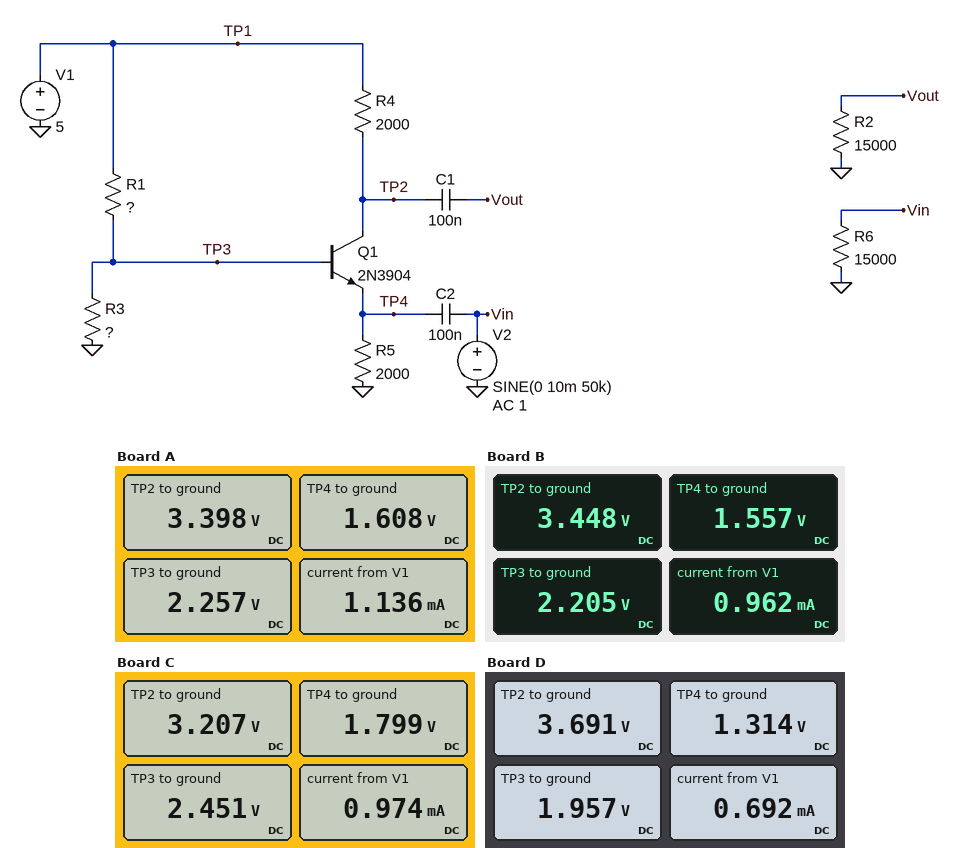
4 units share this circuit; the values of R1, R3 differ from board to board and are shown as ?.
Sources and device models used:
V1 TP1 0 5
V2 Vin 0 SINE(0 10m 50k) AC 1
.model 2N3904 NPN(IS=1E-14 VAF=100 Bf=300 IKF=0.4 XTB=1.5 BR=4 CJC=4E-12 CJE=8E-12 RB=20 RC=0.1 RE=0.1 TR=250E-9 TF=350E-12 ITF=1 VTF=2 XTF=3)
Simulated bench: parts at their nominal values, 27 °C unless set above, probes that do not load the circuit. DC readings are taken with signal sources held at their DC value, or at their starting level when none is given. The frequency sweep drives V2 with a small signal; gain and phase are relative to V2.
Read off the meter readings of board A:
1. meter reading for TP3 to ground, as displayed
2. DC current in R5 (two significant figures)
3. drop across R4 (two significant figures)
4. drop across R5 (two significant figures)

2.257 V
800 µA
1.6 V
1.6 V
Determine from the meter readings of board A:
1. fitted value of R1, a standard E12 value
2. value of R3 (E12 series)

8.2 kΩ
6.8 kΩ
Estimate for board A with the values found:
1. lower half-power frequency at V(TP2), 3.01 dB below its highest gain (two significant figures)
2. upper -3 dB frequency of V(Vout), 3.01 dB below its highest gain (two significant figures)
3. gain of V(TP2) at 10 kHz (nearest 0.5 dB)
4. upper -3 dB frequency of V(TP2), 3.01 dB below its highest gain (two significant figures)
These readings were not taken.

32 kHz
350 kHz
20.5 dB
350 kHz
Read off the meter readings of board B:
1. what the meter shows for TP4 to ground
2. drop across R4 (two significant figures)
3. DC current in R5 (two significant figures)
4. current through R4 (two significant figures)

1.557 V
1.6 V
780 µA
780 µA
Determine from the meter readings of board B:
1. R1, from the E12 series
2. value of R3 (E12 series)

15 kΩ
12 kΩ
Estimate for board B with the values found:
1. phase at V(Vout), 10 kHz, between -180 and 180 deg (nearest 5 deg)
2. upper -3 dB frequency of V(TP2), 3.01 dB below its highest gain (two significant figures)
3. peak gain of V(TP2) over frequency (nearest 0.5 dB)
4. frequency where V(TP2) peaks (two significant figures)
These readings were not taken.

70 deg
250 kHz
30.0 dB
81 kHz
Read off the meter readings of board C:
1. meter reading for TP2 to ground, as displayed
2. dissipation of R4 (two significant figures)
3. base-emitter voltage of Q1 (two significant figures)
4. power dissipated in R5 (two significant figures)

3.207 V
1.6 mW
650 mV
1.6 mW
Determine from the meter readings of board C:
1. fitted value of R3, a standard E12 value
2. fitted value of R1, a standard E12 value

33 kΩ
33 kΩ
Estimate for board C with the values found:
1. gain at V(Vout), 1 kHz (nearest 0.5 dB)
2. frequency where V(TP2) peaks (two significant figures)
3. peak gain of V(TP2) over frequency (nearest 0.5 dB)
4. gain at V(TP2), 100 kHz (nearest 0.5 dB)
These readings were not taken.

0.5 dB
50 kHz
26.0 dB
25.0 dB
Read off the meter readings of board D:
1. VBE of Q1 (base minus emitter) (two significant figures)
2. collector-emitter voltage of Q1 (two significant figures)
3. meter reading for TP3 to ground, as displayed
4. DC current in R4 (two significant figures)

640 mV
2.4 V
1.957 V
650 µA
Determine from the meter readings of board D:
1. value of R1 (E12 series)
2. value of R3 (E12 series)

82 kΩ
56 kΩ
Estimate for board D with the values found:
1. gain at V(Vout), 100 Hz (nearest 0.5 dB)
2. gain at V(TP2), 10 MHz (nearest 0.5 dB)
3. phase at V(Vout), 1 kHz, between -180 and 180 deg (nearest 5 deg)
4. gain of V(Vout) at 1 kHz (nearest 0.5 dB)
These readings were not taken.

-22.5 dB
-1.5 dB
90 deg
0 dB
